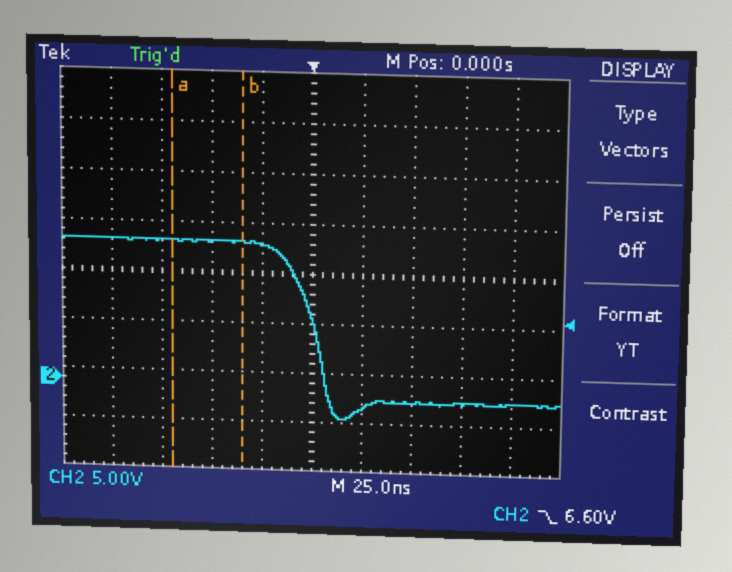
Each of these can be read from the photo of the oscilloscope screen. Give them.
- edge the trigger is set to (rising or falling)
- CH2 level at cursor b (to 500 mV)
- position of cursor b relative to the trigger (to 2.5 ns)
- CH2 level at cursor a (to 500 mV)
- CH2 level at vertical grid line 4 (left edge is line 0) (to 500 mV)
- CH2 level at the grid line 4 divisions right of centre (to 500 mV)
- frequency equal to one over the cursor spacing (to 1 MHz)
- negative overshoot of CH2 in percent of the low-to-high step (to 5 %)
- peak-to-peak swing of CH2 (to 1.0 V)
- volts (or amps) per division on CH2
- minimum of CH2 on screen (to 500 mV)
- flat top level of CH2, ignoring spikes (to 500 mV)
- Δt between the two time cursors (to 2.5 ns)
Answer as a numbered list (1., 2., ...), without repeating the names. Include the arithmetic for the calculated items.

1. falling
2. 14.0 V
3. -35.0 ns
4. 14.0 V
5. 14.0 V
6. -1.5 V
7. 1 / 35.0 ns ≈ 29 MHz
8. 10 %
9. 18.0 V
10. 5 V
11. -3.5 V
12. 14.0 V
13. 35.0 ns
